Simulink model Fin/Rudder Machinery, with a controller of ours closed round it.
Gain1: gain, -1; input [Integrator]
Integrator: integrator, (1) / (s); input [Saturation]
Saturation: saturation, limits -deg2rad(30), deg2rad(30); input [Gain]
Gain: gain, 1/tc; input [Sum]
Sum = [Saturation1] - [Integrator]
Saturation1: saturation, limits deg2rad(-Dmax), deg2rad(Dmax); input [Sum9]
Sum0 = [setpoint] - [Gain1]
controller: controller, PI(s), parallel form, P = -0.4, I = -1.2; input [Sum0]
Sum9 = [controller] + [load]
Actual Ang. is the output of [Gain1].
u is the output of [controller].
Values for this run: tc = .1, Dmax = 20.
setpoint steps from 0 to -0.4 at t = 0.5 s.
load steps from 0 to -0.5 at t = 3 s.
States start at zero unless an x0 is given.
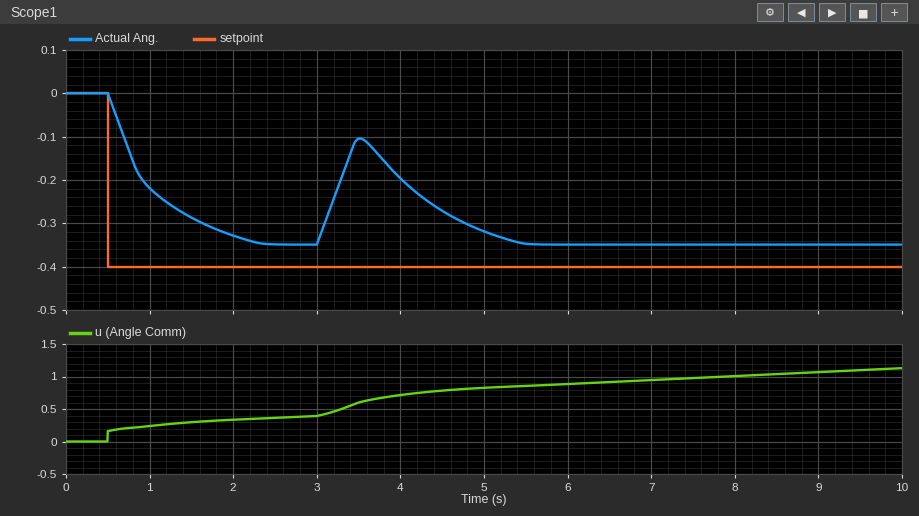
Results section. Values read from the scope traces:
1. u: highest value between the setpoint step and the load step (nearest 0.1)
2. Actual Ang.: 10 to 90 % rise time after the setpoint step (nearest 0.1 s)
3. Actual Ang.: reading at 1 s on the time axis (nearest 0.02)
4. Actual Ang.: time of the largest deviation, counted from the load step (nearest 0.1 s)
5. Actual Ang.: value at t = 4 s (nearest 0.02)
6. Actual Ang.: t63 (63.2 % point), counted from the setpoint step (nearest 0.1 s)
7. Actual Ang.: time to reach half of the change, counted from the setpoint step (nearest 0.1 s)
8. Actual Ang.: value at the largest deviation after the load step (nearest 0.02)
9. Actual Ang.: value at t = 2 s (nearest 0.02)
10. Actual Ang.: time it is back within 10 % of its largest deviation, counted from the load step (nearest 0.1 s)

0.4
1.2 s
-0.22
0.5 s
-0.20
0.5 s
0.3 s
-0.10
-0.32
2.1 s
